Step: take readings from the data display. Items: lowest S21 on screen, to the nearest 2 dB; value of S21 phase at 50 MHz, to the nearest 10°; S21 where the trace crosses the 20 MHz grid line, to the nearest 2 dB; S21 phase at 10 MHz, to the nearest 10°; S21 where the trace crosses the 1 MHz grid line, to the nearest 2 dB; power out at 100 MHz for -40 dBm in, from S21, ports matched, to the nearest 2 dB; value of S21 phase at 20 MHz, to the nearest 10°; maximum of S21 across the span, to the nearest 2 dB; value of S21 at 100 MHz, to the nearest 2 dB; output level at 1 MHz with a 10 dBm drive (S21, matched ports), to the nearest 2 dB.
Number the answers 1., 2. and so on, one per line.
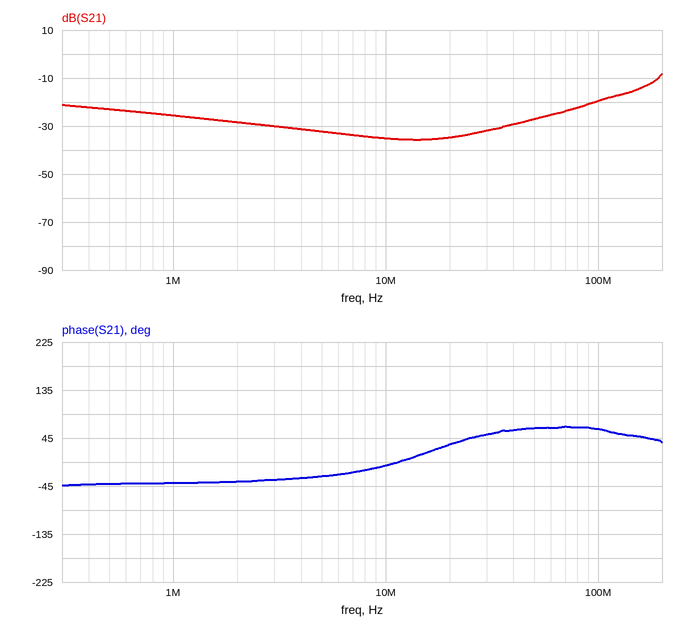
1. -36 dB
2. 60°
3. -34 dB
4. -10°
5. -26 dB
6. -60 dBm
7. 30°
8. -8 dB
9. -20 dB
10. -16 dBm
